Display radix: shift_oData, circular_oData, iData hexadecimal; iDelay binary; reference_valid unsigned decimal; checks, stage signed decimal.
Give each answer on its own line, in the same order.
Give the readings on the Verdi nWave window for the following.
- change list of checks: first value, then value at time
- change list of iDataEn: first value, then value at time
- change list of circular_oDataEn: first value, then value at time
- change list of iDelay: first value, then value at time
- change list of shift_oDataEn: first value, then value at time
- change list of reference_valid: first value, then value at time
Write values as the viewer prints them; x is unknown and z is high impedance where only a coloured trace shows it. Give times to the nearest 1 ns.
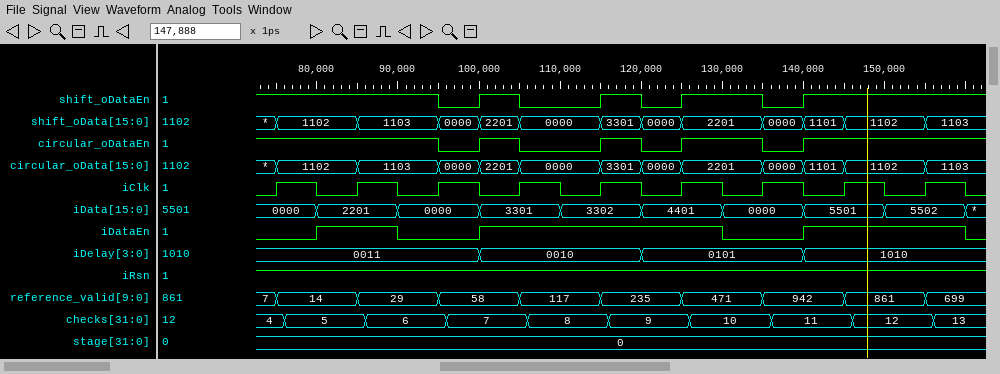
4, 5 at 76 ns, 6 at 86 ns, 7 at 96 ns, 8 at 106 ns, 9 at 116 ns, 10 at 126 ns, 11 at 136 ns, 12 at 146 ns, 13 at 156 ns
0, 1 at 80 ns, 0 at 90 ns, 1 at 100 ns, 0 at 130 ns, 1 at 140 ns, 0 at 160 ns
1, 0 at 95 ns, 1 at 100 ns, 0 at 105 ns, 1 at 115 ns, 0 at 120 ns, 1 at 125 ns, 0 at 135 ns, 1 at 140 ns
0011, 0010 at 100 ns, 0101 at 120 ns, 1010 at 140 ns
1, 0 at 95 ns, 1 at 100 ns, 0 at 105 ns, 1 at 115 ns, 0 at 120 ns, 1 at 125 ns, 0 at 135 ns, 1 at 140 ns
7, 14 at 75 ns, 29 at 85 ns, 58 at 95 ns, 117 at 105 ns, 235 at 115 ns, 471 at 125 ns, 942 at 135 ns, 861 at 145 ns, 699 at 155 ns
